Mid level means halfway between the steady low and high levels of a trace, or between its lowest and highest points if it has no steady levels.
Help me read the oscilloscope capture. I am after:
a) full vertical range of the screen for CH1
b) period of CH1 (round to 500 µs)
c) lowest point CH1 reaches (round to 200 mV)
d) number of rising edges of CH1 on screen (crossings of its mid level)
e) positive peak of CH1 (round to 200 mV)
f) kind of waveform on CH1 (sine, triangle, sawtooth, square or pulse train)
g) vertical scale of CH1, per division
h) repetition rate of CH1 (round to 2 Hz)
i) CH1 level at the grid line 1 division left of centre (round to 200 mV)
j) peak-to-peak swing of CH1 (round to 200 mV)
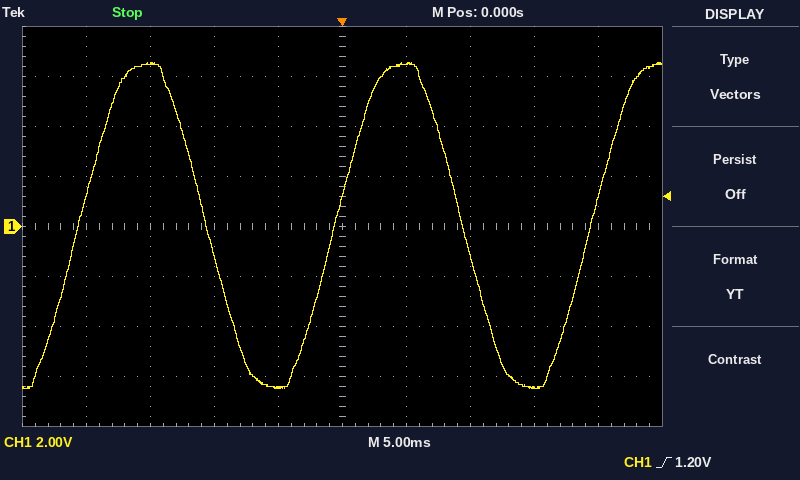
16 V
20.0 ms
-6.4 V
3
6.6 V
sine
2 V
50 Hz
-6.4 V
13.0 V
